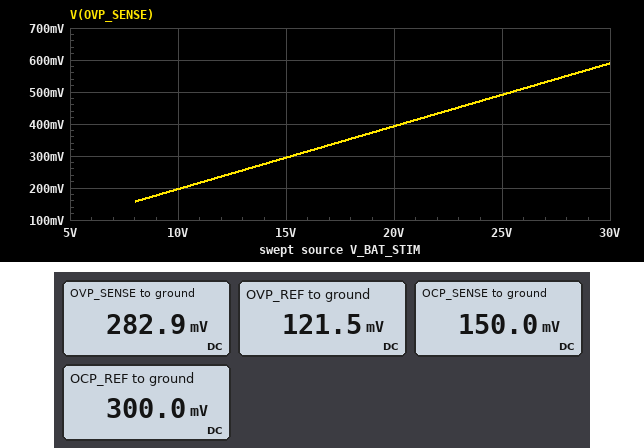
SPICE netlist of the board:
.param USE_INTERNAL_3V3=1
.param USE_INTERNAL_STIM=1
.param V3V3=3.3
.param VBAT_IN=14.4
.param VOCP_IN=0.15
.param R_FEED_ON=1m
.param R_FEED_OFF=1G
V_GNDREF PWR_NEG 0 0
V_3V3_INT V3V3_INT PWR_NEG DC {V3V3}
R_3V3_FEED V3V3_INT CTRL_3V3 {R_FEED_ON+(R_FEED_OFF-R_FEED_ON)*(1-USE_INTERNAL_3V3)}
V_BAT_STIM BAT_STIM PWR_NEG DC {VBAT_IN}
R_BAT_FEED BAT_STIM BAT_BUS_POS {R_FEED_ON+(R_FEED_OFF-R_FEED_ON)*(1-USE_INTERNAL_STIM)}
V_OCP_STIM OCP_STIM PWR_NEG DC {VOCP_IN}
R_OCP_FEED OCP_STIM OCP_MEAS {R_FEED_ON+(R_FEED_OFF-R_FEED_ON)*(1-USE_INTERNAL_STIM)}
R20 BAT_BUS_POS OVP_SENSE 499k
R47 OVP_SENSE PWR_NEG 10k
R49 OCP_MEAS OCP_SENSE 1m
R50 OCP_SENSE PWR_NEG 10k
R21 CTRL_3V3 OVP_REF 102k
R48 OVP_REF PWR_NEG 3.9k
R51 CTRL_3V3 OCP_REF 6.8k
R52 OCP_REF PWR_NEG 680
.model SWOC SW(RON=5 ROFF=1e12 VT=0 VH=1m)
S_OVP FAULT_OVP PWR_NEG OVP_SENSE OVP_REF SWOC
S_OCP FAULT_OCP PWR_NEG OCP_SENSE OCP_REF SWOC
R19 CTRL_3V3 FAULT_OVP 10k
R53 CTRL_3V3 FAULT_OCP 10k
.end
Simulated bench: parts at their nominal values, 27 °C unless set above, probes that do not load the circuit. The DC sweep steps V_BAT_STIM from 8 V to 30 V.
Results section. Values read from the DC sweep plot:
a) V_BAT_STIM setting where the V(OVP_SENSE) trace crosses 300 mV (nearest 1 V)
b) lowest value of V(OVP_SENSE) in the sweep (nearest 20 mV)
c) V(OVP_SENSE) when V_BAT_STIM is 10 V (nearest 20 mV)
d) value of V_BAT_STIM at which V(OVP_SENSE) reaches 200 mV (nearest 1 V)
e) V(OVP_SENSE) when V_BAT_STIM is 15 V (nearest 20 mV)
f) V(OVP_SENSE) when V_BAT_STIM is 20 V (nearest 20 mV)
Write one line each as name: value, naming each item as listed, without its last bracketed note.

V_BAT_STIM setting where the V(OVP_SENSE) trace crosses 300 mV: 15 V
lowest value of V(OVP_SENSE) in the sweep: 160 mV
V(OVP_SENSE) when V_BAT_STIM is 10 V: 200 mV
value of V_BAT_STIM at which V(OVP_SENSE) reaches 200 mV: 10 V
V(OVP_SENSE) when V_BAT_STIM is 15 V: 300 mV
V(OVP_SENSE) when V_BAT_STIM is 20 V: 400 mV
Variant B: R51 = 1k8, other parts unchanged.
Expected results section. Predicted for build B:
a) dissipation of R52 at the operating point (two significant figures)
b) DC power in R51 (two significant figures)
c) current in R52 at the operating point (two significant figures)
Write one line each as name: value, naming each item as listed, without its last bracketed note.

dissipation of R52 at the operating point: 1.2 mW
DC power in R51: 3.2 mW
current in R52 at the operating point: 1.3 mA
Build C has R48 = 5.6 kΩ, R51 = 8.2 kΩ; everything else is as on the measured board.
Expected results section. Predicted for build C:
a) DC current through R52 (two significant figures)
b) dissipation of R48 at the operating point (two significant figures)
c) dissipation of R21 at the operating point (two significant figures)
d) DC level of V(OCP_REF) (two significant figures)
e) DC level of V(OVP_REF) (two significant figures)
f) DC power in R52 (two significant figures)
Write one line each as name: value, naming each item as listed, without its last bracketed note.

DC current through R52: 370 µA
dissipation of R48 at the operating point: 5.3 µW
dissipation of R21 at the operating point: 96 µW
DC level of V(OCP_REF): 250 mV
DC level of V(OVP_REF): 170 mV
DC power in R52: 94 µW
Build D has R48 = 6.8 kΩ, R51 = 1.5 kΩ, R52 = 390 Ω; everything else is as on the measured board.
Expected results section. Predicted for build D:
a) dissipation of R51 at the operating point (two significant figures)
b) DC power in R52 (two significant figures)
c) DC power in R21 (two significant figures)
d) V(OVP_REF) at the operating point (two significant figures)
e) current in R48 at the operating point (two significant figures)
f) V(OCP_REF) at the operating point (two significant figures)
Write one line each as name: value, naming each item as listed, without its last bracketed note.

dissipation of R51 at the operating point: 4.6 mW
DC power in R52: 1.2 mW
DC power in R21: 94 µW
V(OVP_REF) at the operating point: 210 mV
current in R48 at the operating point: 30 µA
V(OCP_REF) at the operating point: 680 mV
